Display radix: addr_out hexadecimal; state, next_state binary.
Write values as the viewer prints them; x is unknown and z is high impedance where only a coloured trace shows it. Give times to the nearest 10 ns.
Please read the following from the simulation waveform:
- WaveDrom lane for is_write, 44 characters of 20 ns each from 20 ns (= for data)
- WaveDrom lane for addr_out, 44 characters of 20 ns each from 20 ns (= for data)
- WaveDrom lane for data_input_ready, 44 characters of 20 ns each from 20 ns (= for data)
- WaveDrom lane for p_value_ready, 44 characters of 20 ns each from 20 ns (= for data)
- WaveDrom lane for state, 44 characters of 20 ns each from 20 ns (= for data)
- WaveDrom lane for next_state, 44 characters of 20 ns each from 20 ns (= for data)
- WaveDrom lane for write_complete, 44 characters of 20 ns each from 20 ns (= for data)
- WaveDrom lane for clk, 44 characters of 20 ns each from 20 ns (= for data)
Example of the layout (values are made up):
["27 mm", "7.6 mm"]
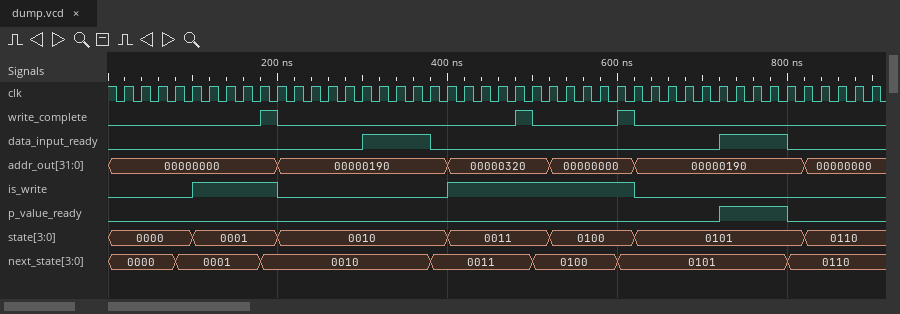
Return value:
["{name: 'is_write', wave: '0...1....0.........1..........0.............'}", "{name: 'addr_out', wave: '=........=.........=.....=....=.........=...', data: '00000000 00000190 00000320 00000000 00000190 00000000'}", "{name: 'data_input_ready', wave: '0.............1...0................1...0....'}", "{name: 'p_value_ready', wave: '0..................................1...0....'}", "{name: 'state', wave: '=...=....=.........=.....=....=.........=...', data: '0000 0001 0010 0011 0100 0101 0110'}", "{name: 'next_state', wave: '=..=....=.........=.....=....=.........=....', data: '0000 0001 0010 0011 0100 0101 0110'}", "{name: 'write_complete', wave: '0.......10.............10....10.............'}", "{name: 'clk', wave: 'p...........................................'}"]
